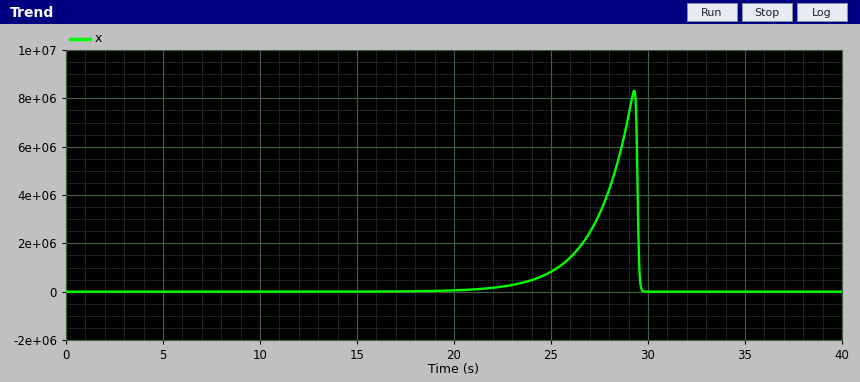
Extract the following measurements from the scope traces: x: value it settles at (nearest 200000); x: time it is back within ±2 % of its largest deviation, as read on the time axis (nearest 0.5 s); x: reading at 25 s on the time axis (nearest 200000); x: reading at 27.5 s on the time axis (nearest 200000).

0
29.5 s
800000
3200000
